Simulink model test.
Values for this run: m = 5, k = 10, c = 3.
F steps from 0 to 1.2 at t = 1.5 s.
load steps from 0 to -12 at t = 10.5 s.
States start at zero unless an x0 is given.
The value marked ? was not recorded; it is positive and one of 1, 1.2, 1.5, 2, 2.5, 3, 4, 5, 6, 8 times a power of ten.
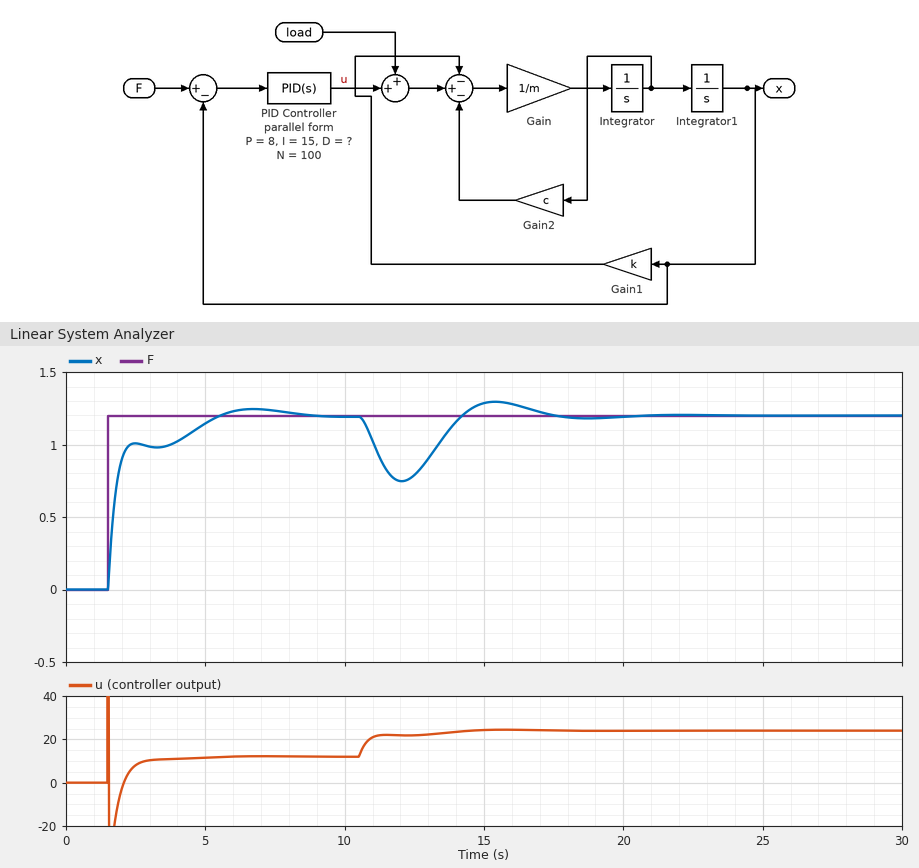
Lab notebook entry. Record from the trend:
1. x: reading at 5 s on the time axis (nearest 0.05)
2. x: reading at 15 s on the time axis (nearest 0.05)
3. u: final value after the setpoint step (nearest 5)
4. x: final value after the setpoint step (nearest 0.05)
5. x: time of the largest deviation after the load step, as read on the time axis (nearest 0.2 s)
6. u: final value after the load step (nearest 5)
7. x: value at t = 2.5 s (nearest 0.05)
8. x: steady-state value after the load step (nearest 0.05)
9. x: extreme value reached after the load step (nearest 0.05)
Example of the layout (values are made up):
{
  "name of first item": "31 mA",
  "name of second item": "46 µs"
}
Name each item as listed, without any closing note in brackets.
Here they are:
{
  "x: reading at 5 s on the time axis": "1.15",
  "x: reading at 15 s on the time axis": "1.30",
  "u: final value after the setpoint step": "10",
  "x: final value after the setpoint step": "1.20",
  "x: time of the largest deviation after the load step, as read on the time axis": "12.0 s",
  "u: final value after the load step": "25",
  "x: value at t = 2.5 s": "1.00",
  "x: steady-state value after the load step": "1.20",
  "x: extreme value reached after the load step": "0.75"
}
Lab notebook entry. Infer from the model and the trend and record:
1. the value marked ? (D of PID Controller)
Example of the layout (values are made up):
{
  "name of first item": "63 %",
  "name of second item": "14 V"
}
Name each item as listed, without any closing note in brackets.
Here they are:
{
  "the value marked ?": "15"
}
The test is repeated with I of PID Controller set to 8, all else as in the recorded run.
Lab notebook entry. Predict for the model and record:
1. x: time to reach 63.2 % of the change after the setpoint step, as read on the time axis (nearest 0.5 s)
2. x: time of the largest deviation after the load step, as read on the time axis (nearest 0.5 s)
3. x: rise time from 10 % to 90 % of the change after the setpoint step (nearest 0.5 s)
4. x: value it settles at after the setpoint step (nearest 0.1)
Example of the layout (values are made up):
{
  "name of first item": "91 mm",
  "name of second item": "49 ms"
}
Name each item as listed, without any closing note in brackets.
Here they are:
{
  "x: time to reach 63.2 % of the change after the setpoint step, as read on the time axis": "2.0 s",
  "x: time of the largest deviation after the load step, as read on the time axis": "12.5 s",
  "x: rise time from 10 % to 90 % of the change after the setpoint step": "4.5 s",
  "x: value it settles at after the setpoint step": "1.2"
}
